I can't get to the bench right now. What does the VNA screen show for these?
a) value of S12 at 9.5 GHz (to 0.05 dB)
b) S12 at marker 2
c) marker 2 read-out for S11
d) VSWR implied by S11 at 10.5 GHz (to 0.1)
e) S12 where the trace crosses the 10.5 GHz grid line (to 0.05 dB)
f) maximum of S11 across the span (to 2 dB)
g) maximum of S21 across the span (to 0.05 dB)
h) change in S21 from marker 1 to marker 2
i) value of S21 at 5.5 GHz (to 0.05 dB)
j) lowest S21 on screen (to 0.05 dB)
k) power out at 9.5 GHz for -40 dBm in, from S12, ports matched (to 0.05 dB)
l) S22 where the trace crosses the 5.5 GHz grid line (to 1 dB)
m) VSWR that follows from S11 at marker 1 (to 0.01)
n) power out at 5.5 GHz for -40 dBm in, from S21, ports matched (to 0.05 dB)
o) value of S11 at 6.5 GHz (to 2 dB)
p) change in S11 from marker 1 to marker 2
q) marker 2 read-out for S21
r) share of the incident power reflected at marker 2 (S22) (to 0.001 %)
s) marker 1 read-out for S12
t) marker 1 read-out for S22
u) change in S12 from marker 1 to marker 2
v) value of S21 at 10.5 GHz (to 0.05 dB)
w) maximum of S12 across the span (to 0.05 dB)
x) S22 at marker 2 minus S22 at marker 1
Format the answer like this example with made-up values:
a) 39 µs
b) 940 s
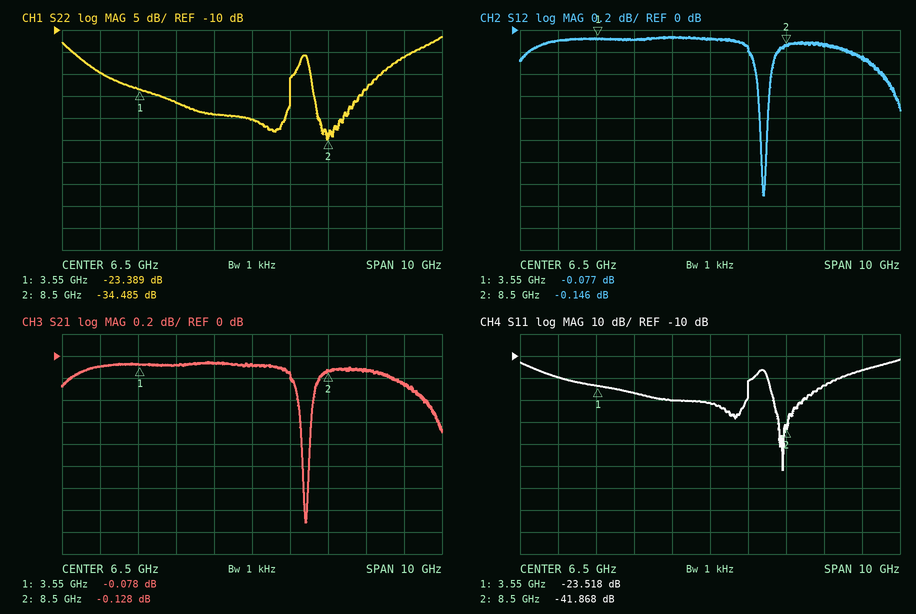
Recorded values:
a) -0.15 dB
b) -0.146 dB
c) -41.868 dB
d) 1.4
e) -0.25 dB
f) -12 dB
g) -0.05 dB
h) -0.050 dB
i) -0.05 dB
j) -1.50 dB
k) -40.15 dBm
l) -29 dB
m) 1.14
n) -40.05 dBm
o) -32 dB
p) -18.350 dB
q) -0.128 dB
r) 0.036 %
s) -0.077 dB
t) -23.389 dB
u) -0.069 dB
v) -0.25 dB
w) -0.05 dB
x) -11.096 dB
